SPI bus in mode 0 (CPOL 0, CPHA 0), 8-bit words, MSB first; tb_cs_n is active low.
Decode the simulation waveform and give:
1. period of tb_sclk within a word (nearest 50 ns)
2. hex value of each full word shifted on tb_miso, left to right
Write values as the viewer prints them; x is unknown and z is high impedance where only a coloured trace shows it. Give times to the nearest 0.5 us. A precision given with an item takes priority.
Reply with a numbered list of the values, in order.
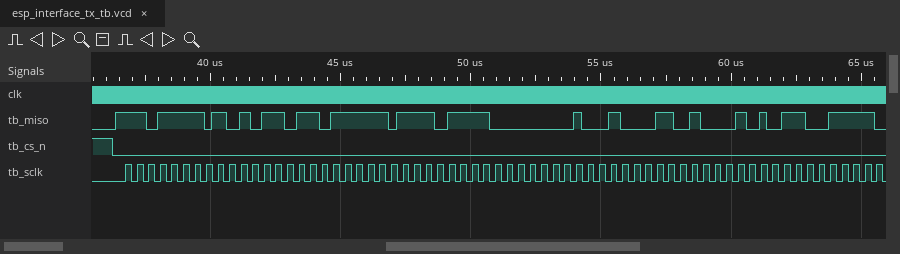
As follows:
1. 450 ns
2. DE, AD, BE, EF, 01, 23, 45, 67
